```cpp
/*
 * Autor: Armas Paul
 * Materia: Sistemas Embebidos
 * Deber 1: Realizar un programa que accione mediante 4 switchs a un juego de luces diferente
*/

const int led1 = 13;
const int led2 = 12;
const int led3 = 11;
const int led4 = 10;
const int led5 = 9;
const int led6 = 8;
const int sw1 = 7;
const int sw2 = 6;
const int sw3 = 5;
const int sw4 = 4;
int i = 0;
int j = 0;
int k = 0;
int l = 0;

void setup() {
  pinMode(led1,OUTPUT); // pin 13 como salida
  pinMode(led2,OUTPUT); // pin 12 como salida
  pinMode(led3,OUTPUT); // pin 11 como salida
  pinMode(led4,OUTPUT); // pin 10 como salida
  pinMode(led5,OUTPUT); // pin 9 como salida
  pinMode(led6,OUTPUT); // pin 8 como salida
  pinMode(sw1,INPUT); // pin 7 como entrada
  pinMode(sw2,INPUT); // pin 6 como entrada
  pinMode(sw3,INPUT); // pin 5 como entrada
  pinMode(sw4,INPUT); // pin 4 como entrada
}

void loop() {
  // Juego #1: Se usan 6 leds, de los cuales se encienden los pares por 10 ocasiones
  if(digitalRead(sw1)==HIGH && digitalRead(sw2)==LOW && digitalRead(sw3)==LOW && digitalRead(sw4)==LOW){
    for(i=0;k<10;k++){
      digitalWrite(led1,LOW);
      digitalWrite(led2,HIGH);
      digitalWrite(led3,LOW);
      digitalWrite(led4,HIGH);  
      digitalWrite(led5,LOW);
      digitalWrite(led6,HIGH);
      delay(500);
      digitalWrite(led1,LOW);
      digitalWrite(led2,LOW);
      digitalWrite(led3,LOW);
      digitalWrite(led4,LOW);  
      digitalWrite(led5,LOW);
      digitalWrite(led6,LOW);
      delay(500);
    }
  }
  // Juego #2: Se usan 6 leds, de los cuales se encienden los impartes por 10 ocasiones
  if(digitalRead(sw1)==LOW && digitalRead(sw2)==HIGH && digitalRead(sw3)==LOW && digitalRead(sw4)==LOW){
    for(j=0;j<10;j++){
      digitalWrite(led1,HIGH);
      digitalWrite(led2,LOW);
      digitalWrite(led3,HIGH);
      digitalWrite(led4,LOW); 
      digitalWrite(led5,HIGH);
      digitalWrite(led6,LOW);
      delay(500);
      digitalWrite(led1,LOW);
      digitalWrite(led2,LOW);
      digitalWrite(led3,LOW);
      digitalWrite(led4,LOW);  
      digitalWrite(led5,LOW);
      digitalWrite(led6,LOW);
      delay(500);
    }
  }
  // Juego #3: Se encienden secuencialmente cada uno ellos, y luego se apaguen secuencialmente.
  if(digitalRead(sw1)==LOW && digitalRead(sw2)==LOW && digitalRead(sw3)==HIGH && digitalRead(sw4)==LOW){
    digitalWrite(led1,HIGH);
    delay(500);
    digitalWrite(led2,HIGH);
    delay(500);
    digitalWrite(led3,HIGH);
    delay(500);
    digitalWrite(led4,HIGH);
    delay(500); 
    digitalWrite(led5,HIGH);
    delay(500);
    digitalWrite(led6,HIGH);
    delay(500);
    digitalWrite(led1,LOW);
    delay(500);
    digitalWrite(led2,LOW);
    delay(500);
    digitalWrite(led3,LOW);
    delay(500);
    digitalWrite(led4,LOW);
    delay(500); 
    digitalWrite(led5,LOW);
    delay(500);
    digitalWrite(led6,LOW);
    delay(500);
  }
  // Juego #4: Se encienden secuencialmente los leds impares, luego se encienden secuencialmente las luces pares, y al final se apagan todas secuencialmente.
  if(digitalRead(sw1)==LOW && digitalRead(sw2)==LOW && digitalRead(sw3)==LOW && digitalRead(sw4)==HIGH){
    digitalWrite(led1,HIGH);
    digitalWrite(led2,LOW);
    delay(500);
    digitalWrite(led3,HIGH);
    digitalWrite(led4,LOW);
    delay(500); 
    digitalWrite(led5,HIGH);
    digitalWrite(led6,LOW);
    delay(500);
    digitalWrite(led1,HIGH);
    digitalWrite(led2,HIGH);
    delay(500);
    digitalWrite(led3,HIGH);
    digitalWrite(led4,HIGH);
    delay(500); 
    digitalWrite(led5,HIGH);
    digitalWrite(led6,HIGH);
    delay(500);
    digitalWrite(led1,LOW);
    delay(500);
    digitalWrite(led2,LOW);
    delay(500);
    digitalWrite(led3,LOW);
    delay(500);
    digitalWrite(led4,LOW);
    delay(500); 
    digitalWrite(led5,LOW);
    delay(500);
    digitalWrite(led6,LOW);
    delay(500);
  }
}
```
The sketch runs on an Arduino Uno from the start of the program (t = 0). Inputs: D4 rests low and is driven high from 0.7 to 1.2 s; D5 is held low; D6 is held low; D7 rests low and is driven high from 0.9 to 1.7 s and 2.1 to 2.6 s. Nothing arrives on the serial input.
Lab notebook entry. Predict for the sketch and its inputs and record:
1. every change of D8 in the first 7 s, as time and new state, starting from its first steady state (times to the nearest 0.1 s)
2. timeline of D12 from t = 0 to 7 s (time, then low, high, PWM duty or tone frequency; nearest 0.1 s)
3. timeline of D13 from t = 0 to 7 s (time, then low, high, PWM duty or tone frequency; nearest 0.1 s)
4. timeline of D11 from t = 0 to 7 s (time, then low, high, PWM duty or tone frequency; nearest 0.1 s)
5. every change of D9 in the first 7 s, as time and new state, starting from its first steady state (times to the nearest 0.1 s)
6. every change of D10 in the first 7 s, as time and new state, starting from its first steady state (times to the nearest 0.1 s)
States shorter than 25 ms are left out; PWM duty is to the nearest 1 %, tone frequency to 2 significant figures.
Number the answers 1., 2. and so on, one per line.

1. 0 s low; 3.2 s high; 6.2 s low
2. 0 s low; 2.2 s high; 4.2 s low
3. 0 s low; 0.7 s high; 3.7 s low
4. 0 s low; 1.2 s high; 4.7 s low
5. 0 s low; 1.7 s high; 5.7 s low
6. 0 s low; 2.7 s high; 5.2 s low
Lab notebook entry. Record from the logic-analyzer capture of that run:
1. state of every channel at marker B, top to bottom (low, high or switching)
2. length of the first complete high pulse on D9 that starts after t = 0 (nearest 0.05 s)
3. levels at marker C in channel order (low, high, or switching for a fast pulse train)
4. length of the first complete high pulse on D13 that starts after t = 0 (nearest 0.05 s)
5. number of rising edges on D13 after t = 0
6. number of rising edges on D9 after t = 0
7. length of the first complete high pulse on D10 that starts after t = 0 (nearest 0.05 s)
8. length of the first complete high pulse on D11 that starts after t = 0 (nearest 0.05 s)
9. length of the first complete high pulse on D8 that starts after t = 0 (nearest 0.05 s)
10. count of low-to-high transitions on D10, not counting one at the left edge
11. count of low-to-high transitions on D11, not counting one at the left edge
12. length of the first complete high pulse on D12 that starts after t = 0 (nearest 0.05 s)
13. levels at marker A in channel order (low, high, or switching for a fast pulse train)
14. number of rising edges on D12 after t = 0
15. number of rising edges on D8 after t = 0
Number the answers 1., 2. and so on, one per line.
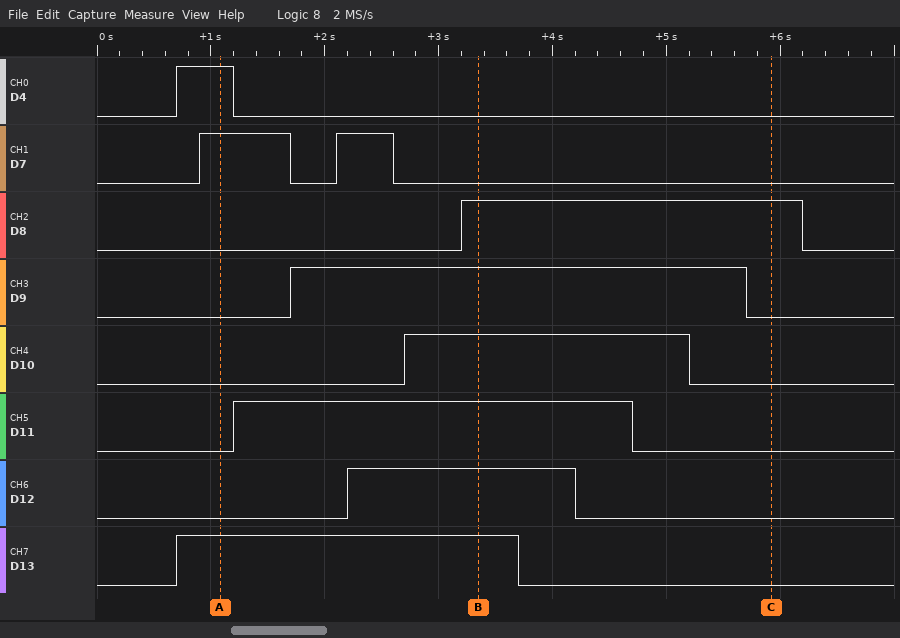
1. D4 low, D7 low, D8 high, D9 high, D10 high, D11 high, D12 high, D13 high
2. 4.00 s
3. D4 low, D7 low, D8 high, D9 low, D10 low, D11 low, D12 low, D13 low
4. 3.00 s
5. 1
6. 1
7. 2.50 s
8. 3.50 s
9. 3.00 s
10. 1
11. 1
12. 2.00 s
13. D4 high, D7 high, D8 low, D9 low, D10 low, D11 low, D12 low, D13 high
14. 1
15. 1
